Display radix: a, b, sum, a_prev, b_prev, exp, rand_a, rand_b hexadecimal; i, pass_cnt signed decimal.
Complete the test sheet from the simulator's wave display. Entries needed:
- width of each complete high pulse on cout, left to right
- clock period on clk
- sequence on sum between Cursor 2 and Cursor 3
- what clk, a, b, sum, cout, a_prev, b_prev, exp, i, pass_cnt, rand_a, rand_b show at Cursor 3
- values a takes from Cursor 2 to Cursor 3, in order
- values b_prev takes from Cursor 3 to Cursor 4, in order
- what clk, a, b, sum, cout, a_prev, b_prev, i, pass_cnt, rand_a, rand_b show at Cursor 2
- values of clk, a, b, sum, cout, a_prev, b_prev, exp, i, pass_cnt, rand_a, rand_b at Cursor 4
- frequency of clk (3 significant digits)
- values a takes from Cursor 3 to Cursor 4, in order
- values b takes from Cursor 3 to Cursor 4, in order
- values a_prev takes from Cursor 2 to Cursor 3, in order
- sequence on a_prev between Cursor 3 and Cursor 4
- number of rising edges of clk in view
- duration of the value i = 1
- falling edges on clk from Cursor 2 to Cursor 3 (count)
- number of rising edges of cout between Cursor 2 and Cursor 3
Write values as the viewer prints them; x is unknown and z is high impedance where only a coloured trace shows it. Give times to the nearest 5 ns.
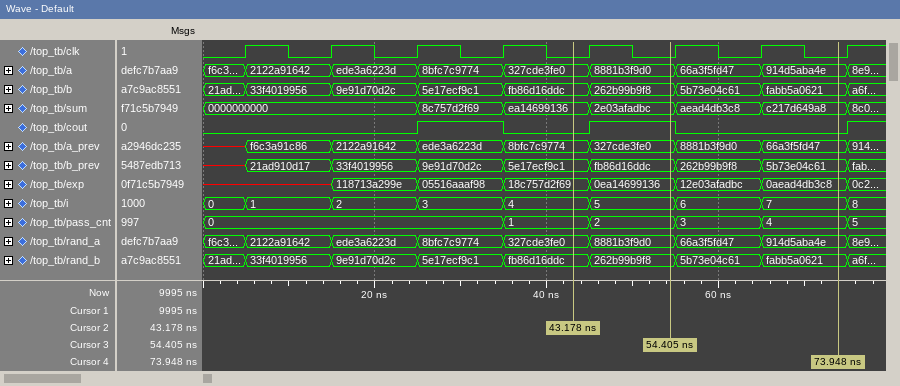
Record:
10 ns, 10 ns
10 ns
ea14699136, 2e03afadbc
clk=0, a=8881b3f9d0, b=262b99b9f8, sum=2e03afadbc, cout=1, a_prev=327cde3fe0, b_prev=fb86d16ddc, exp=0ea14699136, i=5, pass_cnt=2, rand_a=8881b3f9d0, rand_b=262b99b9f8
327cde3fe0, 8881b3f9d0
fb86d16ddc, 262b99b9f8, 5b73e04c61
clk=0, a=327cde3fe0, b=fb86d16ddc, sum=ea14699136, cout=0, a_prev=8bfc7c9774, b_prev=5e17ecf9c1, i=4, pass_cnt=1, rand_a=327cde3fe0, rand_b=fb86d16ddc
clk=0, a=914d5aba4e, b=fabb5a0621, sum=c217d649a8, cout=0, a_prev=66a3f5fd47, b_prev=5b73e04c61, exp=0aead4db3c8, i=7, pass_cnt=4, rand_a=914d5aba4e, rand_b=fabb5a0621
100 MHz
8881b3f9d0, 66a3f5fd47, 914d5aba4e
262b99b9f8, 5b73e04c61, fabb5a0621
8bfc7c9774, 327cde3fe0
327cde3fe0, 8881b3f9d0, 66a3f5fd47
8
10 ns
1
1
